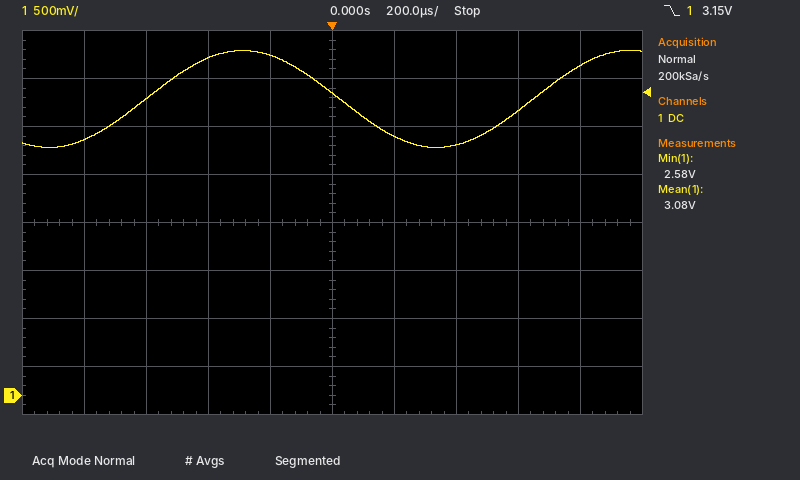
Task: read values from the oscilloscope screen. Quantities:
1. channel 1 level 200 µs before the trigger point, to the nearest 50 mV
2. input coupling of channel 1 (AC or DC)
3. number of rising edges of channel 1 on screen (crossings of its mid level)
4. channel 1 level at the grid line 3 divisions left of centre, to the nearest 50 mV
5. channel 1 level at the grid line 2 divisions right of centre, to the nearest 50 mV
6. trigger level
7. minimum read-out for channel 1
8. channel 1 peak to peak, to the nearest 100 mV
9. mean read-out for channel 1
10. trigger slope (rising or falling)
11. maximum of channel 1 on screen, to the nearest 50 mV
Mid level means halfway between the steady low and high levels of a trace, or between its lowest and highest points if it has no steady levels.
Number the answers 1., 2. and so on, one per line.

1. 3.55 V
2. DC
3. 2
4. 3.10 V
5. 2.60 V
6. 3.15 V
7. 2.58 V
8. 1.00 V
9. 3.08 V
10. falling
11. 3.60 V
